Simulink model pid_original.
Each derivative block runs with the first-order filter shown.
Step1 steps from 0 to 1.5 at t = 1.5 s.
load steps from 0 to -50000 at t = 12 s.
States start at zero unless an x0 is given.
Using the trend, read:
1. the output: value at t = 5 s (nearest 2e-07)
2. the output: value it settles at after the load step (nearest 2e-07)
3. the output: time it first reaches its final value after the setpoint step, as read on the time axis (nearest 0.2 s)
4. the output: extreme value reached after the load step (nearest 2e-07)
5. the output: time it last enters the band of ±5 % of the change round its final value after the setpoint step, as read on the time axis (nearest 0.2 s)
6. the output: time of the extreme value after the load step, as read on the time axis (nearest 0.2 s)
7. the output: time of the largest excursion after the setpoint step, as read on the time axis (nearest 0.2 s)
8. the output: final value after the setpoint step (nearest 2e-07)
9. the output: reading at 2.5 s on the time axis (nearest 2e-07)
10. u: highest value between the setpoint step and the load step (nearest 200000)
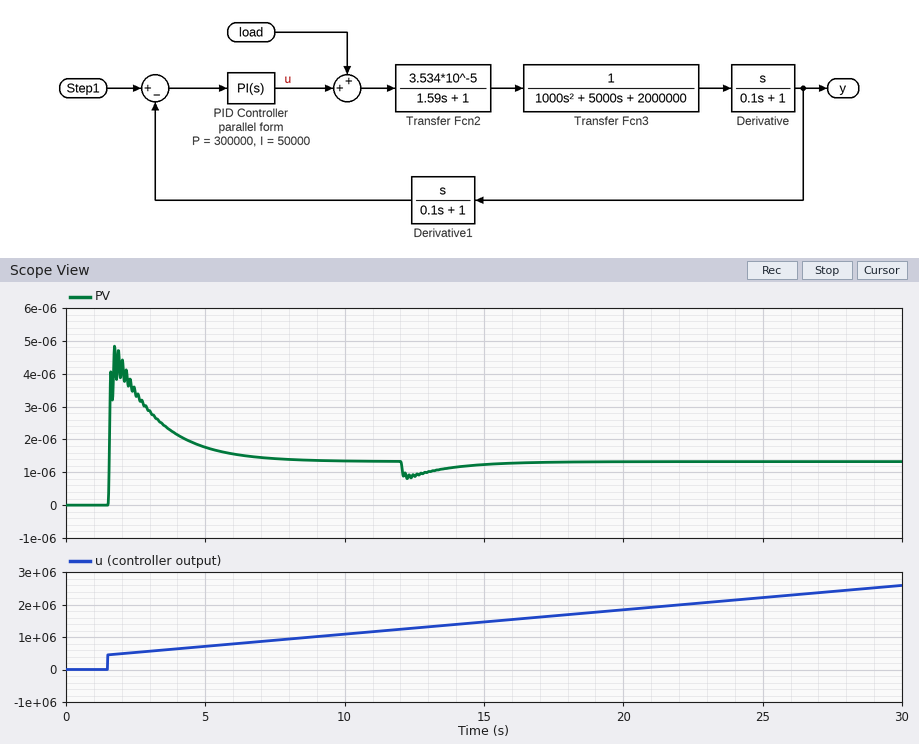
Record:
0.0000018
0.0000014
1.6 s
0.0000008
8.0 s
12.2 s
1.8 s
0.0000014
0.0000034
1200000
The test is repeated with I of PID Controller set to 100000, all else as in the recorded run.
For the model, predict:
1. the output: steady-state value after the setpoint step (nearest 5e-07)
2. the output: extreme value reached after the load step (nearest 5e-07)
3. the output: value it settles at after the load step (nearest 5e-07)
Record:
0.0000025
0.0000020
0.0000025
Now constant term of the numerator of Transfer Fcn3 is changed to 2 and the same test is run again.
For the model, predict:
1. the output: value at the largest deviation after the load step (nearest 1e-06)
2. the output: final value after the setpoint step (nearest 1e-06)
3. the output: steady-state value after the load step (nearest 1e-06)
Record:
0.000002
0.000003
0.000003
